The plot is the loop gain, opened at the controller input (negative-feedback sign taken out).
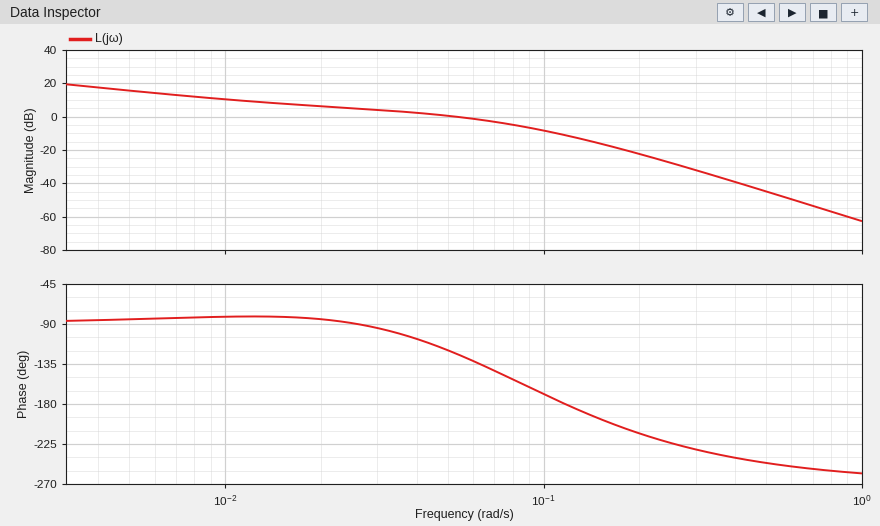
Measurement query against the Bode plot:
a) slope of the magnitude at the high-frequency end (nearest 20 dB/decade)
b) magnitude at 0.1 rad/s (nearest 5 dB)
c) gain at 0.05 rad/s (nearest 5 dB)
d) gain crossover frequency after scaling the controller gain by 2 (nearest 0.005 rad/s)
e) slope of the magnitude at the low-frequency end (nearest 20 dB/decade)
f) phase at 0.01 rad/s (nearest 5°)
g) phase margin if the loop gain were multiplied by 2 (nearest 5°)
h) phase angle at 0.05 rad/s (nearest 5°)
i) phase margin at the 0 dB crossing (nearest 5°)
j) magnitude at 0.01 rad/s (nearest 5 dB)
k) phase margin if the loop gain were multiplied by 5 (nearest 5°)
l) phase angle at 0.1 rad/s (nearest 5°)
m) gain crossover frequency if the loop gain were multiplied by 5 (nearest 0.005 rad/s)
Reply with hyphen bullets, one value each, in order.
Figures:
- -60 dB/decade
- -10 dB
- 0 dB
- 0.085 rad/s
- -20 dB/decade
- -80°
- 20°
- -120°
- 55°
- 10 dB
- -10°
- -170°
- 0.135 rad/s
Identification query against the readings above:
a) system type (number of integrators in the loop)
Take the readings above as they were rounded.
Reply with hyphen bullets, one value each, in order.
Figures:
- 1
